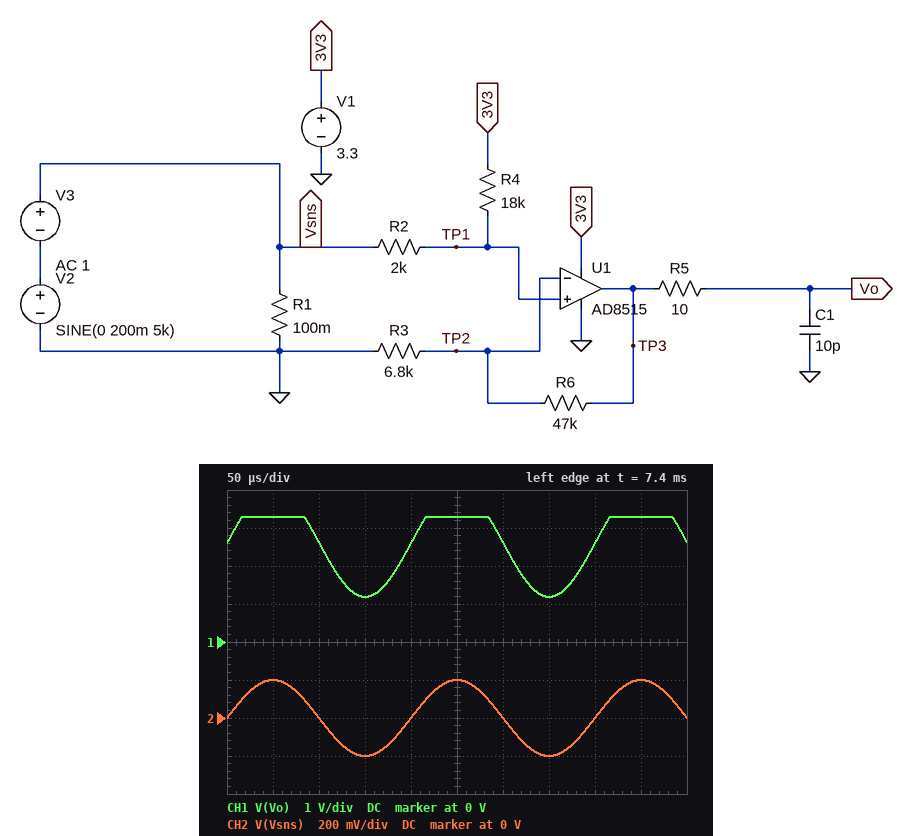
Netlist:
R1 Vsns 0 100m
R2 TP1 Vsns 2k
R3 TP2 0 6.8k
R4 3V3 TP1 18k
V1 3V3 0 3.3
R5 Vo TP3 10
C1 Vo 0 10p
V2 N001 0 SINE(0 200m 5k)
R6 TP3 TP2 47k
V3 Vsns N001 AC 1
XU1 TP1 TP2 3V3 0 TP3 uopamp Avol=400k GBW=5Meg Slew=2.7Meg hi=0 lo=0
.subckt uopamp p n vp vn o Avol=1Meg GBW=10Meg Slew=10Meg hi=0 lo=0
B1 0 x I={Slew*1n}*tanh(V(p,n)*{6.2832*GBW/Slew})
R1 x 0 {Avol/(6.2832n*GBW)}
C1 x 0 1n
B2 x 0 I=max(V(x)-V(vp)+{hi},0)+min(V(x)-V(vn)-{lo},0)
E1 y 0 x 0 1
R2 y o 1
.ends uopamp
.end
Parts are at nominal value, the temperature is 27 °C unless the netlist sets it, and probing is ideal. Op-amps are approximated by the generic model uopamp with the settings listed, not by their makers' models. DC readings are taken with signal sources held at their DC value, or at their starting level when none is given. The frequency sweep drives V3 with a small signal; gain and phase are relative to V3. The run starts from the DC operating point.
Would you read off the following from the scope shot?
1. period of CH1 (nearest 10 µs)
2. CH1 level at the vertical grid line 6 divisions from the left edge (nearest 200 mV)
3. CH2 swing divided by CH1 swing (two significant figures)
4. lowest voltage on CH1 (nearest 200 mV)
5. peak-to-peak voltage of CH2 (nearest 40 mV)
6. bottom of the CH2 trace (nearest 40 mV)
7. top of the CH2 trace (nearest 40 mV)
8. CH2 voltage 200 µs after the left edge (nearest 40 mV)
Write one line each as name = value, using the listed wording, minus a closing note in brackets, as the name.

period of CH1 = 200 µs
CH1 level at the vertical grid line 6 divisions from the left edge = 2.6 V
CH2 swing divided by CH1 swing = 0.19
lowest voltage on CH1 = 1.2 V
peak-to-peak voltage of CH2 = 400 mV
bottom of the CH2 trace = -200 mV
top of the CH2 trace = 200 mV
CH2 voltage 200 µs after the left edge = 0 V
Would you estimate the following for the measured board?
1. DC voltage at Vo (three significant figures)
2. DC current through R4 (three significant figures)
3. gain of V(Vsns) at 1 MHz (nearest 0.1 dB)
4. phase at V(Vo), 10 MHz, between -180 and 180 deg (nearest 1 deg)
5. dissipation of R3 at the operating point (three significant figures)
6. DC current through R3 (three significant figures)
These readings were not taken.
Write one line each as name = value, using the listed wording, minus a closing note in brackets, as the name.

DC voltage at Vo = 2.61 V
DC current through R4 = 165 µA
gain of V(Vsns) at 1 MHz = 0 dB
phase at V(Vo), 10 MHz, between -180 and 180 deg = -87 deg
dissipation of R3 at the operating point = 16.0 µW
DC current through R3 = 48.5 µA
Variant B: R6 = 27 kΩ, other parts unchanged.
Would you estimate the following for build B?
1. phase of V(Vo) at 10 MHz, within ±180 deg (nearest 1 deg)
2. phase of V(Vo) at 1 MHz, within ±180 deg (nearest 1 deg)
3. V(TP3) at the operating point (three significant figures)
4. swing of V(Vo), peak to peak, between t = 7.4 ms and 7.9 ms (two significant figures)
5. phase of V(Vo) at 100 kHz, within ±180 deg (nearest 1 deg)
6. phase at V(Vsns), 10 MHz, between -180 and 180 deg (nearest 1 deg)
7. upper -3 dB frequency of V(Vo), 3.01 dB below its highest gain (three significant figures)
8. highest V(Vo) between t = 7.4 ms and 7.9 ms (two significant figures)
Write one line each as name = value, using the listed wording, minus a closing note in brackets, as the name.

phase of V(Vo) at 10 MHz, within ±180 deg = -85 deg
phase of V(Vo) at 1 MHz, within ±180 deg = -45 deg
V(TP3) at the operating point = 1.64 V
swing of V(Vo), peak to peak, between t = 7.4 ms and 7.9 ms = 1.8 V
phase of V(Vo) at 100 kHz, within ±180 deg = -6 deg
phase at V(Vsns), 10 MHz, between -180 and 180 deg = 0 deg
upper -3 dB frequency of V(Vo), 3.01 dB below its highest gain = 1.01 MHz
highest V(Vo) between t = 7.4 ms and 7.9 ms = 2.5 V
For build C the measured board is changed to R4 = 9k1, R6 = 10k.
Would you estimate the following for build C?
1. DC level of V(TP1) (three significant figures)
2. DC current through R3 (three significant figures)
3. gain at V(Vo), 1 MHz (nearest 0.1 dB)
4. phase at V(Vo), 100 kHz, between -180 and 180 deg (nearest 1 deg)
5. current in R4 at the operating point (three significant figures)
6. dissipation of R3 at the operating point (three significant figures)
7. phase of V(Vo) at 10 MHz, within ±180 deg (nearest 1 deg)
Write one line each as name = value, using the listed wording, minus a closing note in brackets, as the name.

DC level of V(TP1) = 595 mV
DC current through R3 = 87.4 µA
gain at V(Vo), 1 MHz = 5.2 dB
phase at V(Vo), 100 kHz, between -180 and 180 deg = -3 deg
current in R4 at the operating point = 297 µA
dissipation of R3 at the operating point = 52.0 µW
phase of V(Vo) at 10 MHz, within ±180 deg = -79 deg
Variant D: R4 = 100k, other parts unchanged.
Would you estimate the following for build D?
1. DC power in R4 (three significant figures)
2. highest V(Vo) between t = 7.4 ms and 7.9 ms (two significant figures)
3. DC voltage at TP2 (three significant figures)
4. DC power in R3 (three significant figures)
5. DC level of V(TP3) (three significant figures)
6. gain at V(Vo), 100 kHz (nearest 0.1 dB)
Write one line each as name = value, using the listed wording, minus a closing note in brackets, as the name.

DC power in R4 = 105 µW
highest V(Vo) between t = 7.4 ms and 7.9 ms = 2.1 V
DC voltage at TP2 = 64.7 mV
DC power in R3 = 616 nW
DC level of V(TP3) = 512 mV
gain at V(Vo), 100 kHz = 17.7 dB
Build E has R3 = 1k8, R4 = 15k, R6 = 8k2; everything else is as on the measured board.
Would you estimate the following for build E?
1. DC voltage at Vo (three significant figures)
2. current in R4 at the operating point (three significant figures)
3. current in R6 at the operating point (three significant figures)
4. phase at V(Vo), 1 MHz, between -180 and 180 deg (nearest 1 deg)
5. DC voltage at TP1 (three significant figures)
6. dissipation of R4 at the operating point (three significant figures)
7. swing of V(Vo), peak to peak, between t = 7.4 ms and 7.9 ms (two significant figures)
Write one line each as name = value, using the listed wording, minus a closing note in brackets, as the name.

DC voltage at Vo = 2.16 V
current in R4 at the operating point = 194 µA
current in R6 at the operating point = 216 µA
phase at V(Vo), 1 MHz, between -180 and 180 deg = -48 deg
DC voltage at TP1 = 388 mV
dissipation of R4 at the operating point = 565 µW
swing of V(Vo), peak to peak, between t = 7.4 ms and 7.9 ms = 2.0 V
